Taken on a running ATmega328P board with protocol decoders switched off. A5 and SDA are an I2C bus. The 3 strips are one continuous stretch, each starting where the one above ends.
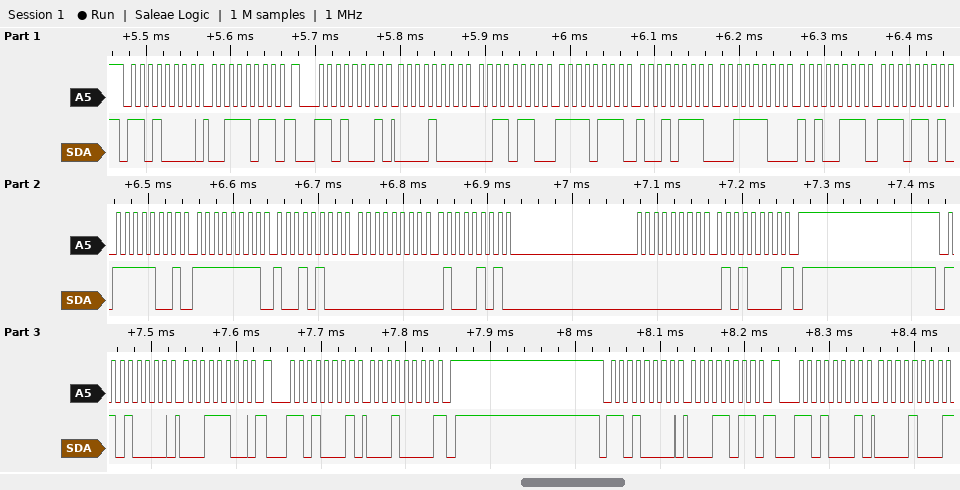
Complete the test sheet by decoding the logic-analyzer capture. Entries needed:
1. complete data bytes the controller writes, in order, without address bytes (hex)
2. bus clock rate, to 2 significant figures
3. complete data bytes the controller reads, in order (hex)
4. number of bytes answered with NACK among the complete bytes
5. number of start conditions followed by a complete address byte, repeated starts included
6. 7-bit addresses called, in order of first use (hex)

3B 1C 1B
100 kHz
08 36 F7 97 3C A7 ED F9 FF 94 00 45 00 50 10 08
3
6
0x68
